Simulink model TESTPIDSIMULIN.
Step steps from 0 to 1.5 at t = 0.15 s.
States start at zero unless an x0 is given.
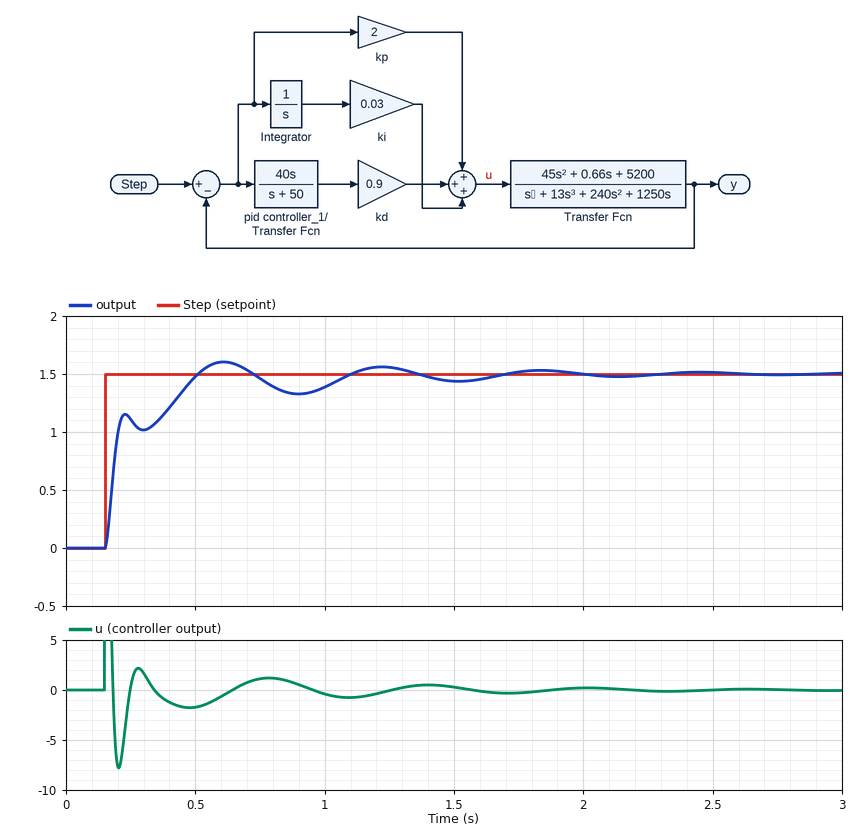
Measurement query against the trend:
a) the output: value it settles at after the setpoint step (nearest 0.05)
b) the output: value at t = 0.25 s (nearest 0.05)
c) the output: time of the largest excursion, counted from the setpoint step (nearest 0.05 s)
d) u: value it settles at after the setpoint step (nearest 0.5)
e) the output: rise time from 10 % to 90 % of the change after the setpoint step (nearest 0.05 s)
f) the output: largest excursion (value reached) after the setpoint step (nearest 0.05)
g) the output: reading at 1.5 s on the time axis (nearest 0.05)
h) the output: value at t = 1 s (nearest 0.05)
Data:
1.50
1.10
0.45 s
0.0
0.30 s
1.60
1.45
1.40
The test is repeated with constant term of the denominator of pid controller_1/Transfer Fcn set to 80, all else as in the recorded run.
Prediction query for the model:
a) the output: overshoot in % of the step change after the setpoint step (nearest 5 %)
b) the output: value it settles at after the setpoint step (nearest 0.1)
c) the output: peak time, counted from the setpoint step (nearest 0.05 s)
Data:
10 %
1.5
0.50 s
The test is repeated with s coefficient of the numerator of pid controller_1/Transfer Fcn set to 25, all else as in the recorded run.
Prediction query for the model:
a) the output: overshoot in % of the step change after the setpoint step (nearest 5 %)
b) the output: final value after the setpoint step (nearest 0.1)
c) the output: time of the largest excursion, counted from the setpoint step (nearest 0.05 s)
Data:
10 %
1.5
0.50 s
